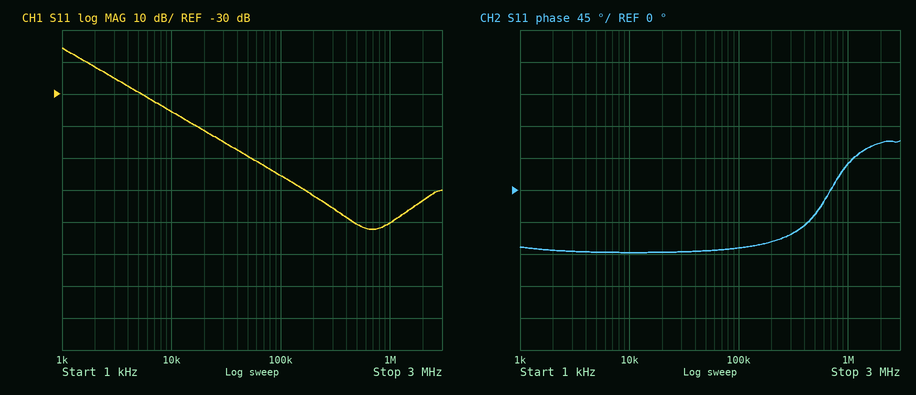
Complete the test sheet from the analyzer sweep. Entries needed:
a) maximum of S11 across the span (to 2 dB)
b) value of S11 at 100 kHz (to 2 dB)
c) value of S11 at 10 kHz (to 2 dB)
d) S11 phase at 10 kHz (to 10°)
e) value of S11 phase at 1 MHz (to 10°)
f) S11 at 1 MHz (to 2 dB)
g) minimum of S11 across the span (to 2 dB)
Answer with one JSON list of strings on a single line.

["-16 dB", "-56 dB", "-36 dB", "-90°", "40°", "-70 dB", "-72 dB"]
